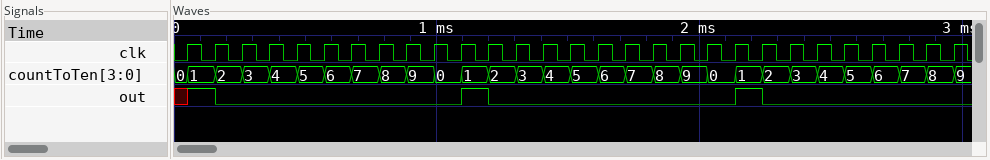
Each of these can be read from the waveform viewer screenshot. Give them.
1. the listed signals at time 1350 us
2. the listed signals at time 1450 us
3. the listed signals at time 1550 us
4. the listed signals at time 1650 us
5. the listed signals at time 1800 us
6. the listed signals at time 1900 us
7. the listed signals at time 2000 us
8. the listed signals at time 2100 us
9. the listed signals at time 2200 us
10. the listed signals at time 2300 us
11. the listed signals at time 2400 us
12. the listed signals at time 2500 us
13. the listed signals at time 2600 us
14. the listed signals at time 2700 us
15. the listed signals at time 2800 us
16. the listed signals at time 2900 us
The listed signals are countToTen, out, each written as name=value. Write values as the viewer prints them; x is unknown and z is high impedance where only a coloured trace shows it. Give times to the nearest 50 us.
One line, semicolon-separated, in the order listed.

countToTen=3, out=0; countToTen=4, out=0; countToTen=5, out=0; countToTen=6, out=0; countToTen=7, out=0; countToTen=8, out=0; countToTen=9, out=0; countToTen=0, out=0; countToTen=1, out=1; countToTen=2, out=0; countToTen=3, out=0; countToTen=4, out=0; countToTen=5, out=0; countToTen=6, out=0; countToTen=7, out=0; countToTen=8, out=0
